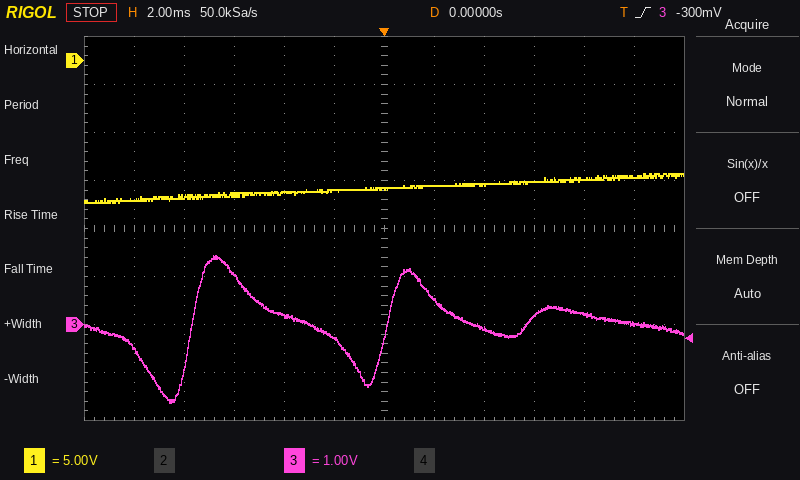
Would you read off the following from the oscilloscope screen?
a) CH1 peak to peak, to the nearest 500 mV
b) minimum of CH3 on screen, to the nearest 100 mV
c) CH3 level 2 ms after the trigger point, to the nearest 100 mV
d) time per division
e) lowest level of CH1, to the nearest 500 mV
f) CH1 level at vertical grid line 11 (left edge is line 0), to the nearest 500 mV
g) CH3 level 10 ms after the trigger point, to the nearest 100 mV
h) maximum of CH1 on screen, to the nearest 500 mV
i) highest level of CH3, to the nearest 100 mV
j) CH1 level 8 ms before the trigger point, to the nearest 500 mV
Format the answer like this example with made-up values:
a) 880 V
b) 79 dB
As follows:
a) 3.0 V
b) -1.6 V
c) 500 mV
d) 2 ms
e) -15.0 V
f) -12.0 V
g) 0.0 V
h) -12.0 V
i) 1.4 V
j) -14.0 V
